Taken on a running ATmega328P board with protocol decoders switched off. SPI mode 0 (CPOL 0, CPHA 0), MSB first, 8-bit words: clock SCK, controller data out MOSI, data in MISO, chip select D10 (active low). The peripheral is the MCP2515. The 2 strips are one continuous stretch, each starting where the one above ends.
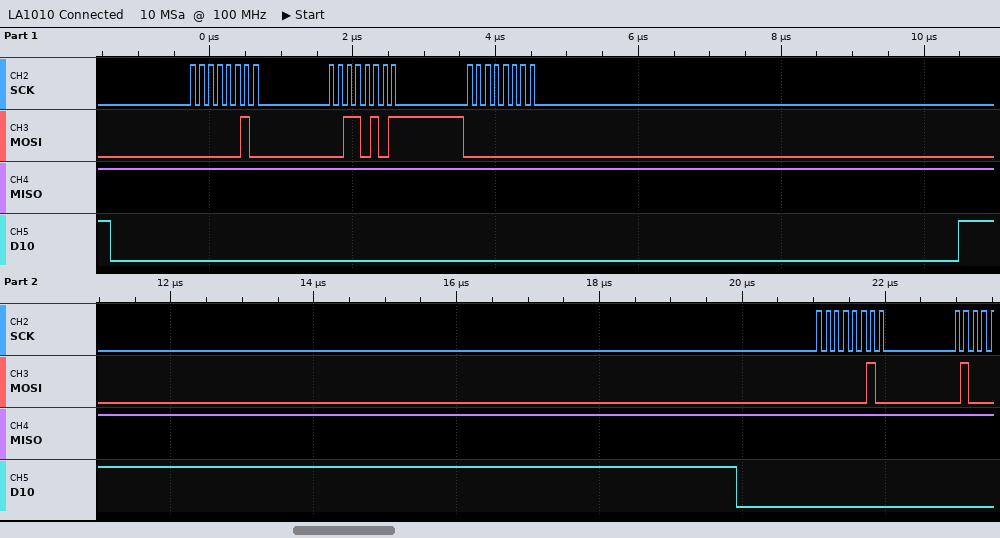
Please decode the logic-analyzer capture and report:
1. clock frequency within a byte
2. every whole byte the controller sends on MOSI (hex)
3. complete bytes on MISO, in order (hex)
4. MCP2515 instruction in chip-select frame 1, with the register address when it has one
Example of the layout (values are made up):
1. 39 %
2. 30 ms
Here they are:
1. 8 MHz
2. 02 35 00 02
3. FF FF FF FF
4. WRITE 0x35
